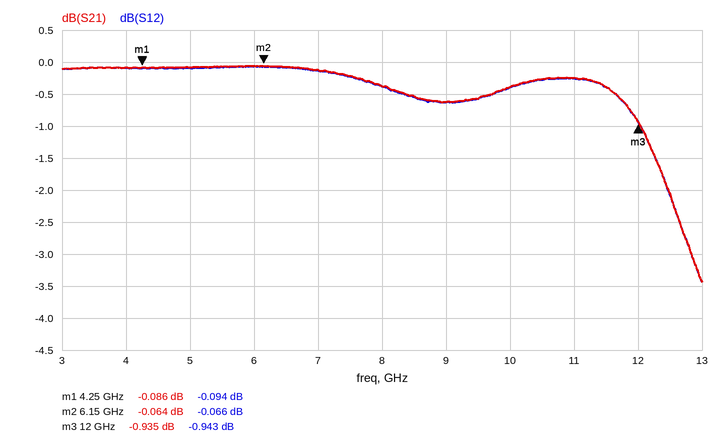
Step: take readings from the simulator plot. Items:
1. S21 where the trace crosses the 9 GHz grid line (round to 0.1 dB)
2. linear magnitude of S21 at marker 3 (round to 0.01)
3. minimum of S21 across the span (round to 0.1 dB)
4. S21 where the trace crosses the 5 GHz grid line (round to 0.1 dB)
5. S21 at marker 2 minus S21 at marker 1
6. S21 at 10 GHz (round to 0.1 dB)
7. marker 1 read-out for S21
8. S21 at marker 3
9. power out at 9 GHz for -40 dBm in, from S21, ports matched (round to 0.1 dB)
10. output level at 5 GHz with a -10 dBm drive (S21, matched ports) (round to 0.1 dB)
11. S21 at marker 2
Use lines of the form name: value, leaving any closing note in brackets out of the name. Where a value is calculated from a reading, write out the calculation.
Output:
S21 where the trace crosses the 9 GHz grid line: -0.6 dB
linear magnitude of S21 at marker 3: 10^(-0.935/20) ≈ 0.90
minimum of S21 across the span: -3.4 dB
S21 where the trace crosses the 5 GHz grid line: -0.1 dB
S21 at marker 2 minus S21 at marker 1: -0.064 − (-0.086) = 0.022 dB
S21 at 10 GHz: -0.4 dB
marker 1 read-out for S21: -0.086 dB
S21 at marker 3: -0.935 dB
power out at 9 GHz for -40 dBm in, from S21, ports matched: -40 dBm + (-0.6 dB) = -40.6 dBm
output level at 5 GHz with a -10 dBm drive (S21, matched ports): -10 dBm + (-0.1 dB) = -10.1 dBm
S21 at marker 2: -0.064 dB
